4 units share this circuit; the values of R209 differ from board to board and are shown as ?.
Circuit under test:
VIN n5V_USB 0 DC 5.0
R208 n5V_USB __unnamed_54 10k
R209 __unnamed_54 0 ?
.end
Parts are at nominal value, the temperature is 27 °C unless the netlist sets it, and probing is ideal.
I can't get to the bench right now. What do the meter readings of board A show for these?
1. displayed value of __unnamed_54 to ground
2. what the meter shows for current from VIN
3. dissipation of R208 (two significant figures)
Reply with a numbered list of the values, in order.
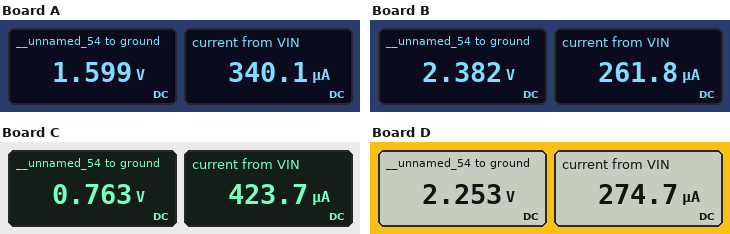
1. 1.599 V
2. 340.1 µA
3. 1.2 mW
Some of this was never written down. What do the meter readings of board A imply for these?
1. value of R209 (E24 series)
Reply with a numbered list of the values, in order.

1. 4.7 kΩ
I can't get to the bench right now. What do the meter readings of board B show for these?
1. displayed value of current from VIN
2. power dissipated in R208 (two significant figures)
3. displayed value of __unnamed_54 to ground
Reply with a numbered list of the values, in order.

1. 261.8 µA
2. 690 µW
3. 2.382 V
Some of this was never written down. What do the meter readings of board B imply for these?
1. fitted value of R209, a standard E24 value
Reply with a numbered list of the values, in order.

1. 9.1 kΩ
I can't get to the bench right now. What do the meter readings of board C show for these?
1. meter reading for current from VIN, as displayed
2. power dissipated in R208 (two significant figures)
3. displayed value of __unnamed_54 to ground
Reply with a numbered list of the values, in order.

1. 423.7 µA
2. 1.8 mW
3. 0.763 V
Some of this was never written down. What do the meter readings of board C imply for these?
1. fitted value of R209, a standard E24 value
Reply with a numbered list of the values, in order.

1. 1.8 kΩ
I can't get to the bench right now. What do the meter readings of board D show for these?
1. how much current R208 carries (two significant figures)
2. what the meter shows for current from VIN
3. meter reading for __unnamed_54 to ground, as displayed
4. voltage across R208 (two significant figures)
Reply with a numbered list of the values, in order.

1. 270 µA
2. 274.7 µA
3. 2.253 V
4. 2.7 V
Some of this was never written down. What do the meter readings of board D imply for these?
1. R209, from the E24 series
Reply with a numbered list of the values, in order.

1. 8.2 kΩ
